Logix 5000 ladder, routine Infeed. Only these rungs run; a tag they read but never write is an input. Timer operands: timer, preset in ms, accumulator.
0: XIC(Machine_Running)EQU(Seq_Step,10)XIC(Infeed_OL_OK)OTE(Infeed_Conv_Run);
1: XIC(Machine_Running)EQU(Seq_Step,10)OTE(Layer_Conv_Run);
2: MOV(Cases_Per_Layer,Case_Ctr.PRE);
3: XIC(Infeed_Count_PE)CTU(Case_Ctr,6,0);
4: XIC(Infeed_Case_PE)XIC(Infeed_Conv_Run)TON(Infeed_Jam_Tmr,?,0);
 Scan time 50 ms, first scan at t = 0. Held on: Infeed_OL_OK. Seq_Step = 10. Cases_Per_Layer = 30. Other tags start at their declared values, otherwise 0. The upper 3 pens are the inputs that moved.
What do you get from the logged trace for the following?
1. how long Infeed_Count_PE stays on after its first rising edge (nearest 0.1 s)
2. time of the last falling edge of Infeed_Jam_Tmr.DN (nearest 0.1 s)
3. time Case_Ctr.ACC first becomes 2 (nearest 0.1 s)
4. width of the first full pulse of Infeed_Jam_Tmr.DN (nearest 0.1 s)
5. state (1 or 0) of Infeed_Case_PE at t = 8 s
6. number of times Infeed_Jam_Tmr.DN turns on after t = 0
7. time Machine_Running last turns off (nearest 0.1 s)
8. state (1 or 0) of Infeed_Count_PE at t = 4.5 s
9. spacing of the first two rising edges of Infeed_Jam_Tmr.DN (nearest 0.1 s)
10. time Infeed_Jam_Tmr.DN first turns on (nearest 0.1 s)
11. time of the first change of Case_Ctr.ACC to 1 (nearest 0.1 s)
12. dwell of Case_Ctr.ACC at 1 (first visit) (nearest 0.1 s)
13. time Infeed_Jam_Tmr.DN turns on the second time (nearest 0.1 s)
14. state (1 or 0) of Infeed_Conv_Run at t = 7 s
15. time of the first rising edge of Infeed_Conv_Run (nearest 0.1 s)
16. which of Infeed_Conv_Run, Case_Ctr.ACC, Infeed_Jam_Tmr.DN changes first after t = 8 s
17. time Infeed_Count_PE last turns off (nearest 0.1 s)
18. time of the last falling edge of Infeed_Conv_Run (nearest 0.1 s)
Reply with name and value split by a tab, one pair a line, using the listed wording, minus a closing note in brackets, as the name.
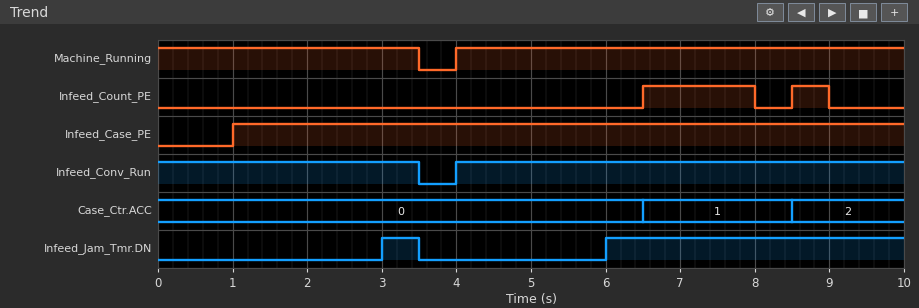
how long Infeed_Count_PE stays on after its first rising edge	1.5 s
time of the last falling edge of Infeed_Jam_Tmr.DN	3.5 s
time Case_Ctr.ACC first becomes 2	8.5 s
width of the first full pulse of Infeed_Jam_Tmr.DN	0.5 s
state (1 or 0) of Infeed_Case_PE at t = 8 s	1
number of times Infeed_Jam_Tmr.DN turns on after t = 0	2
time Machine_Running last turns off	3.5 s
state (1 or 0) of Infeed_Count_PE at t = 4.5 s	0
spacing of the first two rising edges of Infeed_Jam_Tmr.DN	3.0 s
time Infeed_Jam_Tmr.DN first turns on	3.0 s
time of the first change of Case_Ctr.ACC to 1	6.5 s
dwell of Case_Ctr.ACC at 1 (first visit)	2.0 s
time Infeed_Jam_Tmr.DN turns on the second time	6.0 s
state (1 or 0) of Infeed_Conv_Run at t = 7 s	1
time of the first rising edge of Infeed_Conv_Run	4.0 s
which of Infeed_Conv_Run, Case_Ctr.ACC, Infeed_Jam_Tmr.DN changes first after t = 8 s	Case_Ctr.ACC
time Infeed_Count_PE last turns off	9.0 s
time of the last falling edge of Infeed_Conv_Run	3.5 s
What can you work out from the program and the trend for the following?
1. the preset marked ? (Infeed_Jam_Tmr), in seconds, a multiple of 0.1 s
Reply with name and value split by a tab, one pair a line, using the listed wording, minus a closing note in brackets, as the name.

the preset marked ? (Infeed_Jam_Tmr), in seconds, a multiple of 0.1 s	2.0 s
